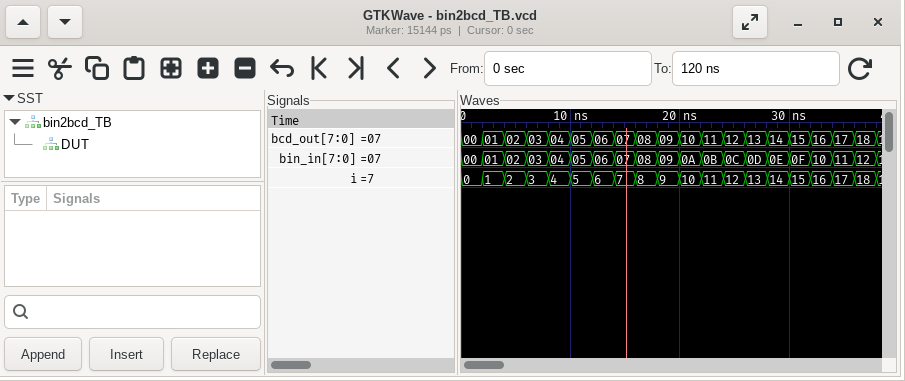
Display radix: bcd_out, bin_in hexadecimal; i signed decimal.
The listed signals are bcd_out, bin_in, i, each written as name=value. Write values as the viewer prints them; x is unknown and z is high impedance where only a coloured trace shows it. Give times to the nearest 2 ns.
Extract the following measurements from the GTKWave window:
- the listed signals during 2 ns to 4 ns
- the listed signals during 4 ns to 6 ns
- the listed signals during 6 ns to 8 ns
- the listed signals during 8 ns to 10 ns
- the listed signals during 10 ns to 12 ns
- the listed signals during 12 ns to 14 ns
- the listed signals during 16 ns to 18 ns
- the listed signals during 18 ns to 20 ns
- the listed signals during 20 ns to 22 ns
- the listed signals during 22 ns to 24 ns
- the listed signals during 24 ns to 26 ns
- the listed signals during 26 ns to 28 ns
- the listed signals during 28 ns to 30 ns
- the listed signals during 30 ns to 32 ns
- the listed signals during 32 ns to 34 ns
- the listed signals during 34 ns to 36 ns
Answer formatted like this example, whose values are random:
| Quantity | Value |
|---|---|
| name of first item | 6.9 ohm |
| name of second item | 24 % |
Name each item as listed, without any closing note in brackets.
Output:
| Quantity | Value |
|---|---|
| the listed signals during 2 ns to 4 ns | bcd_out=01, bin_in=01, i=1 |
| the listed signals during 4 ns to 6 ns | bcd_out=02, bin_in=02, i=2 |
| the listed signals during 6 ns to 8 ns | bcd_out=03, bin_in=03, i=3 |
| the listed signals during 8 ns to 10 ns | bcd_out=04, bin_in=04, i=4 |
| the listed signals during 10 ns to 12 ns | bcd_out=05, bin_in=05, i=5 |
| the listed signals during 12 ns to 14 ns | bcd_out=06, bin_in=06, i=6 |
| the listed signals during 16 ns to 18 ns | bcd_out=08, bin_in=08, i=8 |
| the listed signals during 18 ns to 20 ns | bcd_out=09, bin_in=09, i=9 |
| the listed signals during 20 ns to 22 ns | bcd_out=10, bin_in=0A, i=10 |
| the listed signals during 22 ns to 24 ns | bcd_out=11, bin_in=0B, i=11 |
| the listed signals during 24 ns to 26 ns | bcd_out=12, bin_in=0C, i=12 |
| the listed signals during 26 ns to 28 ns | bcd_out=13, bin_in=0D, i=13 |
| the listed signals during 28 ns to 30 ns | bcd_out=14, bin_in=0E, i=14 |
| the listed signals during 30 ns to 32 ns | bcd_out=15, bin_in=0F, i=15 |
| the listed signals during 32 ns to 34 ns | bcd_out=16, bin_in=10, i=16 |
| the listed signals during 34 ns to 36 ns | bcd_out=17, bin_in=11, i=17 |
